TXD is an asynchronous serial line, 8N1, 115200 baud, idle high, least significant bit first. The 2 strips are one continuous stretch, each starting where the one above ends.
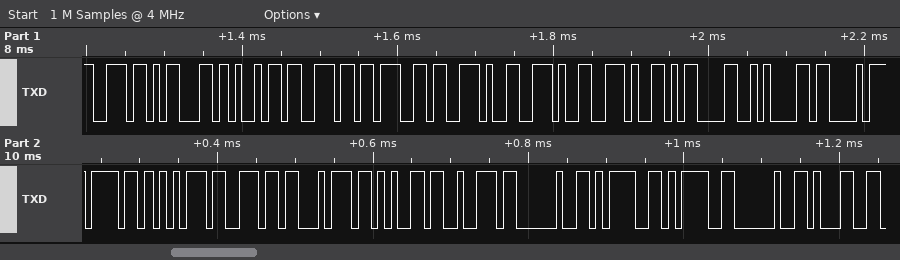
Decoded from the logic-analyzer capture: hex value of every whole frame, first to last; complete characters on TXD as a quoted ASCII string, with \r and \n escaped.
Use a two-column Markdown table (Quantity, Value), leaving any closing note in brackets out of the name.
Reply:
| Quantity | Value |
|---|---|
| hex value of every whole frame, first to last | 6E 63 69 6E 67 2E 2E 2E 0D 0A 43 6F 75 6E 74 65 72 20 3D 3D 20 31 |
| complete characters on TXD as a quoted ASCII string, with \r and \n escaped | "ncing...\r\nCounter == 1" |
